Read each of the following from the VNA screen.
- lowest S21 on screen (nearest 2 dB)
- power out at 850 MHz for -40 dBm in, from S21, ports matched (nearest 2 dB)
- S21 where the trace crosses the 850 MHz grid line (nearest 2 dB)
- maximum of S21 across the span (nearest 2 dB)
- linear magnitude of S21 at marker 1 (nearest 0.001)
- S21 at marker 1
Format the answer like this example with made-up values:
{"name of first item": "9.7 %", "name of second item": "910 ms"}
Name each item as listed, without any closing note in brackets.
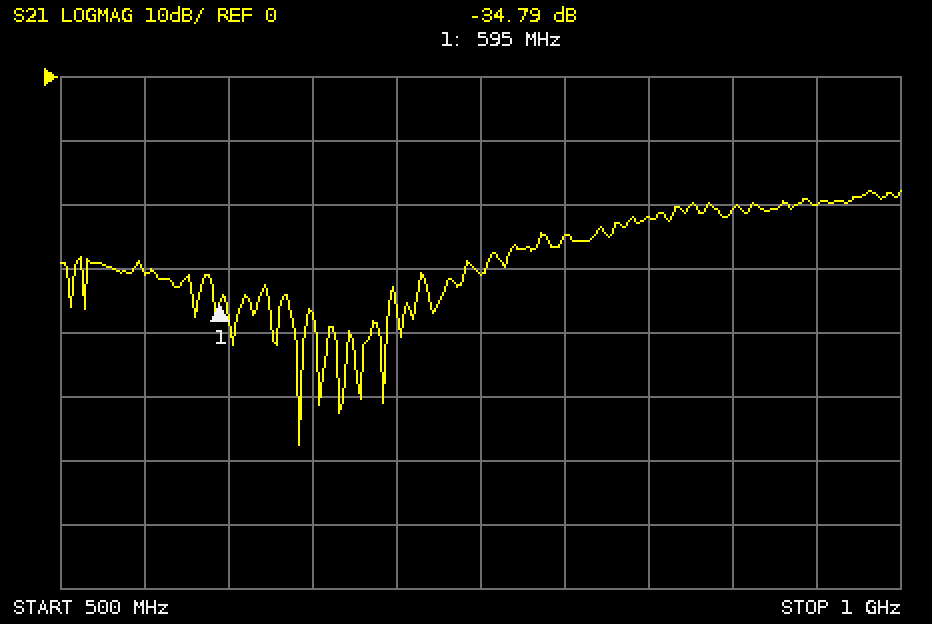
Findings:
{"lowest S21 on screen": "-58 dB", "power out at 850 MHz for -40 dBm in, from S21, ports matched": "-62 dBm", "S21 where the trace crosses the 850 MHz grid line": "-22 dB", "maximum of S21 across the span": "-18 dB", "linear magnitude of S21 at marker 1": "0.018", "S21 at marker 1": "-34.79 dB"}
